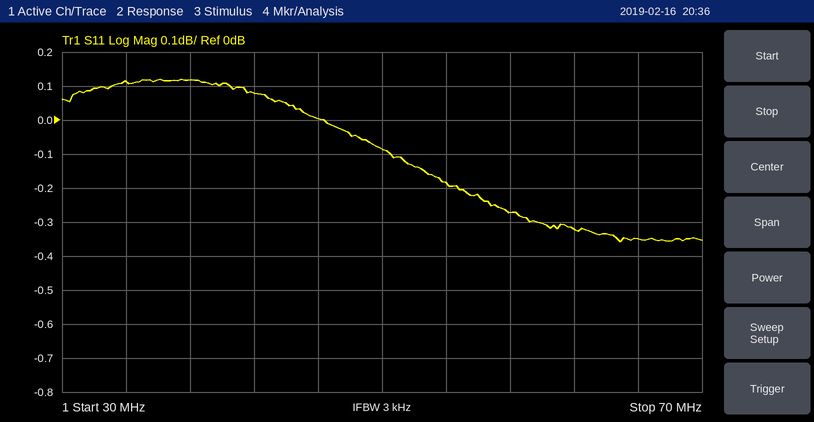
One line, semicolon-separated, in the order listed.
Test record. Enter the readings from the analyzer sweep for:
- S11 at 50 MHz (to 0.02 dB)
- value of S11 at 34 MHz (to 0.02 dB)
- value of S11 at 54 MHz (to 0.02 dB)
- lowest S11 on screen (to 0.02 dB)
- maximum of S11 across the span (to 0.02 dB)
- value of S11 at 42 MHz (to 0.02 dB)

-0.08 dB; 0.12 dB; -0.18 dB; -0.36 dB; 0.12 dB; 0.08 dB
